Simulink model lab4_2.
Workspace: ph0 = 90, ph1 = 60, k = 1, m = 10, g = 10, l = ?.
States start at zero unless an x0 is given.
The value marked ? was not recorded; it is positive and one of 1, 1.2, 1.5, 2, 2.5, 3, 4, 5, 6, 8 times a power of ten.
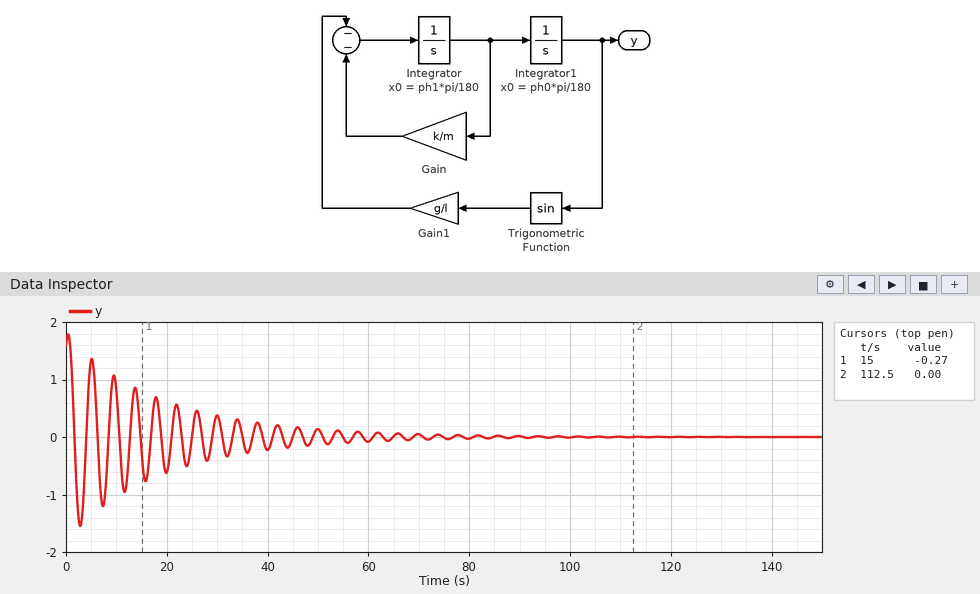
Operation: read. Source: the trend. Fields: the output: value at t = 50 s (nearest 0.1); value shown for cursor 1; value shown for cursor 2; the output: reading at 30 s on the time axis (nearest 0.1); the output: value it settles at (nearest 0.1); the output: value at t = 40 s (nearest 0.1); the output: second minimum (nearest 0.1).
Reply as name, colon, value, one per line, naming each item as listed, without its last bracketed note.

the output: value at t = 50 s: 0.1
value shown for cursor 1: -0.27
value shown for cursor 2: 0.00
the output: reading at 30 s on the time axis: 0.4
the output: value it settles at: 0.0
the output: value at t = 40 s: -0.2
the output: second minimum: -1.2
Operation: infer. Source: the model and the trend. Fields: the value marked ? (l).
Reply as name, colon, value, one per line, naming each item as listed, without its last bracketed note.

the value marked ?: 4
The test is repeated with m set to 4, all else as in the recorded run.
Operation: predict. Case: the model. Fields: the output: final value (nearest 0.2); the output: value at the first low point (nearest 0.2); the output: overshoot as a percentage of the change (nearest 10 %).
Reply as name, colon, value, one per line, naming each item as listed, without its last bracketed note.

the output: final value: 0.0
the output: value at the first low point: -1.2
the output: overshoot as a percentage of the change: 80 %
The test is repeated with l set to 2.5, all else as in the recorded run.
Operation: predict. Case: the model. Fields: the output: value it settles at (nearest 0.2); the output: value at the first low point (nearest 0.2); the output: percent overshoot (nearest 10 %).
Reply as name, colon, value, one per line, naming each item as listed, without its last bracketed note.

the output: value it settles at: 0.0
the output: value at the first low point: -1.6
the output: percent overshoot: 100 %
